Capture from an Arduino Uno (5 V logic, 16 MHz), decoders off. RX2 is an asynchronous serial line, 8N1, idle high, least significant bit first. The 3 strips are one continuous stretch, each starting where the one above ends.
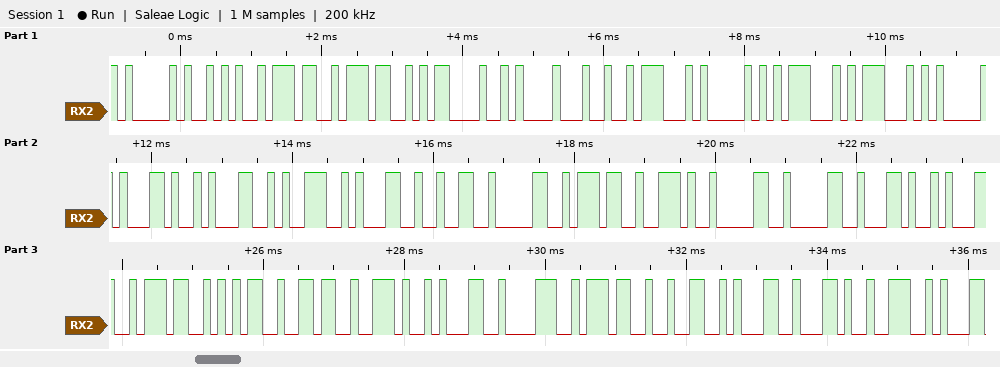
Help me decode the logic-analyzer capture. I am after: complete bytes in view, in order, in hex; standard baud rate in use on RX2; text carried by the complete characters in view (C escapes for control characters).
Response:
41 2A 37 37 0D 0A 24 47 50 47 47 41 2C 31 39 31 32 30 37 2E 30 30 2C 31 37 35 36 2E 31 38 37 32 31 2C 4E
9600 baud
"A*77\r\n$GPGGA,191207.00,1756.18721,N"
